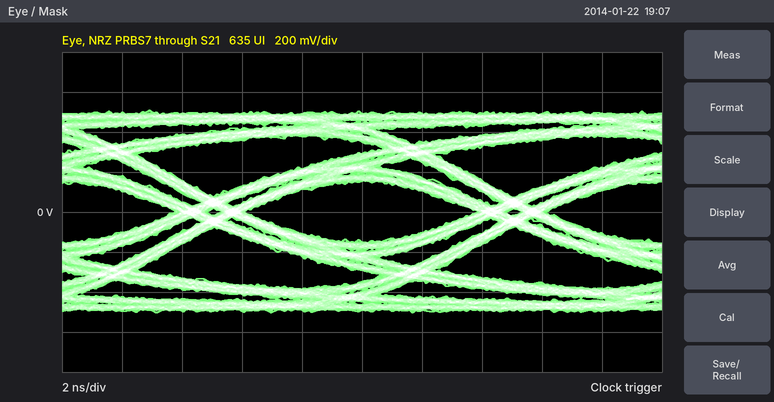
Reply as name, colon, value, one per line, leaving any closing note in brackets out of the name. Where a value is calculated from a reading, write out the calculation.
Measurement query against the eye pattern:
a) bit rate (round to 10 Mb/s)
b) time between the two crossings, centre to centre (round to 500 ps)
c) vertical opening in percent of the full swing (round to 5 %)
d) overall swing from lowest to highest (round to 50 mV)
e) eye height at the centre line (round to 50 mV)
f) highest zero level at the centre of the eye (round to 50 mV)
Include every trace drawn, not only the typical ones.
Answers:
bit rate: 100 Mb/s
time between the two crossings, centre to centre: 10.0 ns
vertical opening in percent of the full swing: 300 mV / 1.00 V ≈ 30 %
overall swing from lowest to highest: 1.00 V
eye height at the centre line: 300 mV
highest zero level at the centre of the eye: -150 mV
